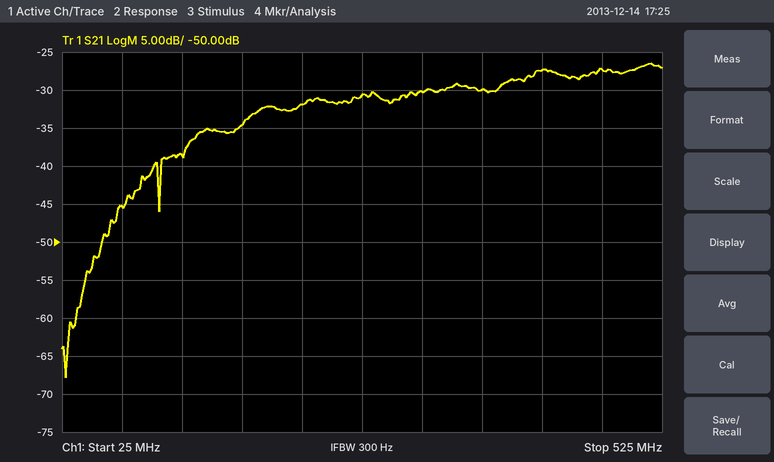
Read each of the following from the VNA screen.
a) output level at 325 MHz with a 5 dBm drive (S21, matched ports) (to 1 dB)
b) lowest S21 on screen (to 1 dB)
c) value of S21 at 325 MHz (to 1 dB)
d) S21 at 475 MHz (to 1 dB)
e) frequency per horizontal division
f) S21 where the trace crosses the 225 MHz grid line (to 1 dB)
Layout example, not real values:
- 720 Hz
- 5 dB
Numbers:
- -25 dBm
- -68 dB
- -30 dB
- -27 dB
- 50 MHz
- -32 dB
